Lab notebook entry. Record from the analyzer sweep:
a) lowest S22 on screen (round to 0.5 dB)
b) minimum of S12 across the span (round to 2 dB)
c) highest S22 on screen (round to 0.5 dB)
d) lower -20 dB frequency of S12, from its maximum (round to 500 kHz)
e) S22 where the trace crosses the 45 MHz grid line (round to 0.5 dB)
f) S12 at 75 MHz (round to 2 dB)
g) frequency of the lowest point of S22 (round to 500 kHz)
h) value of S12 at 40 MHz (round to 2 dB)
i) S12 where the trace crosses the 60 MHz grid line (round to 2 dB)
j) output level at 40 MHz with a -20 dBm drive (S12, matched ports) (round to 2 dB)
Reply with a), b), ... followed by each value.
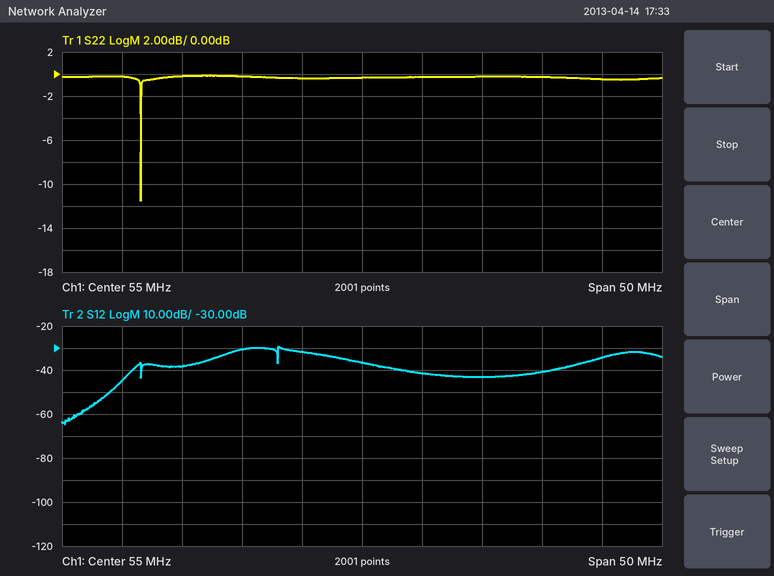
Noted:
a) -11.5 dB
b) -64 dB
c) 0.0 dB
d) 34.0 MHz
e) 0.0 dB
f) -34 dB
g) 36.5 MHz
h) -38 dB
i) -42 dB
j) -58 dBm
